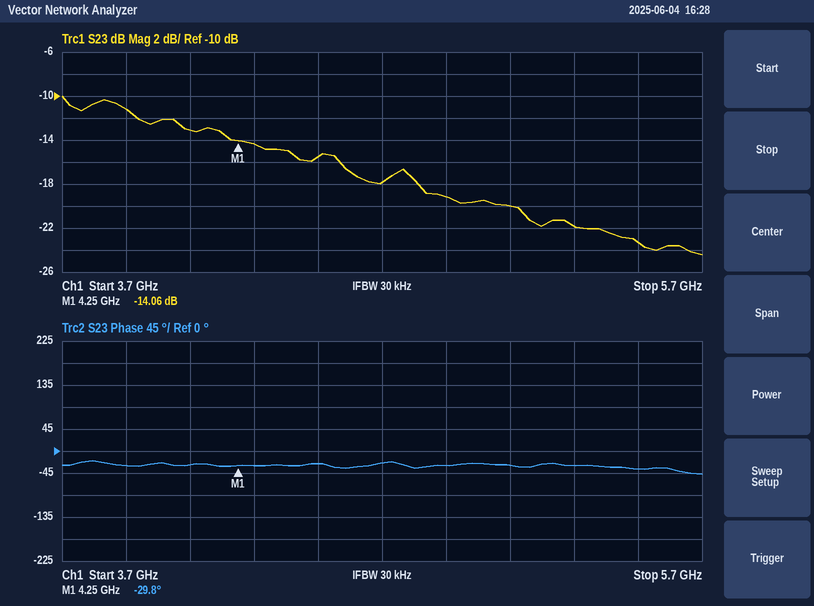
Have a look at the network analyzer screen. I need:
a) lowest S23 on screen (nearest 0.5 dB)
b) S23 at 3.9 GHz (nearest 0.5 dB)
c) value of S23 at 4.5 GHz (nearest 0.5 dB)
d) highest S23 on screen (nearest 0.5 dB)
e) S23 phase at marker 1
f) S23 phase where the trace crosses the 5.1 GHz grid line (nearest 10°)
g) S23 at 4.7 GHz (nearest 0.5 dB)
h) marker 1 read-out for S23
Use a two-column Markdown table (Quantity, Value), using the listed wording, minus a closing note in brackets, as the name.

| Quantity | Value |
|---|---|
| lowest S23 on screen | -24.5 dB |
| S23 at 3.9 GHz | -11.0 dB |
| value of S23 at 4.5 GHz | -15.5 dB |
| highest S23 on screen | -10.0 dB |
| S23 phase at marker 1 | -29.8° |
| S23 phase where the trace crosses the 5.1 GHz grid line | -30° |
| S23 at 4.7 GHz | -18.0 dB |
| marker 1 read-out for S23 | -14.06 dB |
